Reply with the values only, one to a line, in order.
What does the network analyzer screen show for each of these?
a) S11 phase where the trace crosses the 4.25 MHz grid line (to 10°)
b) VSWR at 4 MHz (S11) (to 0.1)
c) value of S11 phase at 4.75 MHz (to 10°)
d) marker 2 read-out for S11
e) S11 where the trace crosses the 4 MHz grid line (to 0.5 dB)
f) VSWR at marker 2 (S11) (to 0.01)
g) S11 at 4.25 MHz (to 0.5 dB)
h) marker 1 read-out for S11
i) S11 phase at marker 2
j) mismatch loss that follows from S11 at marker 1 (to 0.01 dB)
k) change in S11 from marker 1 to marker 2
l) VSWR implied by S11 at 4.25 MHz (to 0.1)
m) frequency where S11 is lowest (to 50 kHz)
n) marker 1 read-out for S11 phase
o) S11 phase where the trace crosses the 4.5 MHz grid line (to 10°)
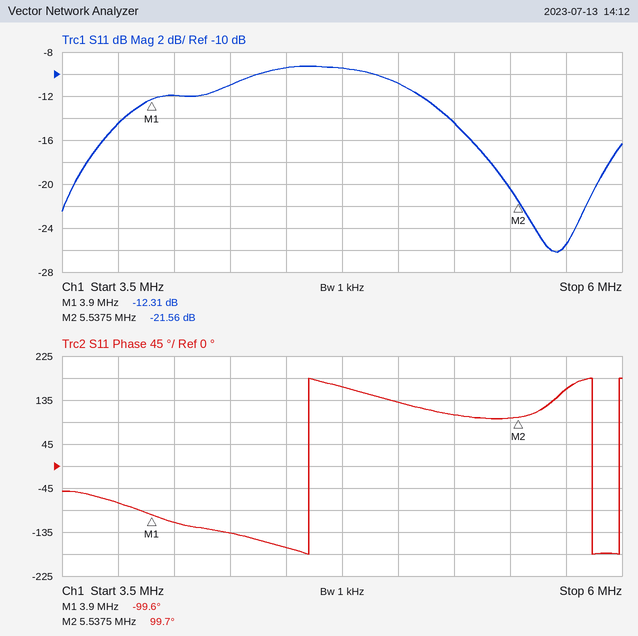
-140°
1.7
160°
-21.56 dB
-12.0 dB
1.18
-11.0 dB
-12.31 dB
99.7°
0.26 dB
-9.25 dB
1.8
5.70 MHz
-99.6°
-170°
